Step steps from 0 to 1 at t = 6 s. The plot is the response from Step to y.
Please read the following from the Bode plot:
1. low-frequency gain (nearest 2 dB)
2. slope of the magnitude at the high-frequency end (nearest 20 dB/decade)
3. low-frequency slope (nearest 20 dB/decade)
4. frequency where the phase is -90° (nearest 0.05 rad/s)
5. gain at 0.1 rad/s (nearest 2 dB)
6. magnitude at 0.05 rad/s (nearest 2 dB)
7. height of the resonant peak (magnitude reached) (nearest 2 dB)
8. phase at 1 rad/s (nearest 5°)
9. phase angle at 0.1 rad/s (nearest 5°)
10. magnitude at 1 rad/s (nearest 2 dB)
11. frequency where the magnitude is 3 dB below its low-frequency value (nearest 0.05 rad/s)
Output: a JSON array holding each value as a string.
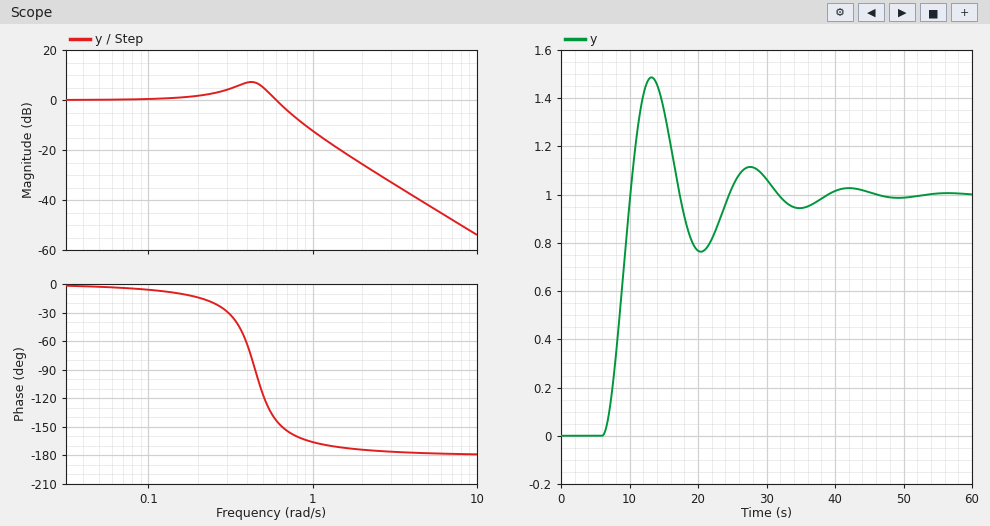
["0 dB", "-40 dB/decade", "0 dB/decade", "0.45 rad/s", "0 dB", "0 dB", "8 dB", "-165°", "-5°", "-12 dB", "0.65 rad/s"]
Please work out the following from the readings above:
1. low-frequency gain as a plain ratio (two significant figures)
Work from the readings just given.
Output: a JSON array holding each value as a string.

["1.0"]
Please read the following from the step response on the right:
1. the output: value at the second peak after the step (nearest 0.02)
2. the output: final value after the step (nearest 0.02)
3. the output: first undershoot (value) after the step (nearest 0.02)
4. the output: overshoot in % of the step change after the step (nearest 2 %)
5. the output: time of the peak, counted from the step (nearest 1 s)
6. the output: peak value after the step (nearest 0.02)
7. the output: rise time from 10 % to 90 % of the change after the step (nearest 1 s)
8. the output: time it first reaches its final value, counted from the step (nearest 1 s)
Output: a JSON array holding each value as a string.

["1.12", "1.00", "0.76", "48 %", "7 s", "1.48", "3 s", "4 s"]
